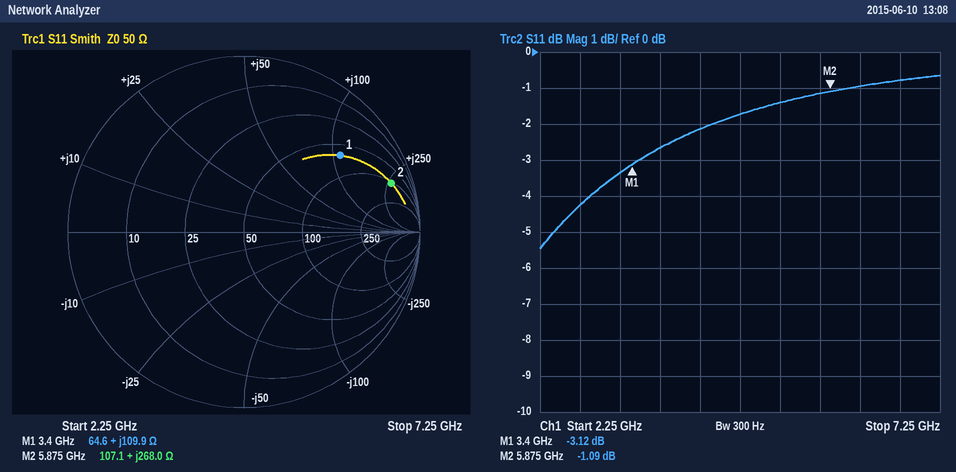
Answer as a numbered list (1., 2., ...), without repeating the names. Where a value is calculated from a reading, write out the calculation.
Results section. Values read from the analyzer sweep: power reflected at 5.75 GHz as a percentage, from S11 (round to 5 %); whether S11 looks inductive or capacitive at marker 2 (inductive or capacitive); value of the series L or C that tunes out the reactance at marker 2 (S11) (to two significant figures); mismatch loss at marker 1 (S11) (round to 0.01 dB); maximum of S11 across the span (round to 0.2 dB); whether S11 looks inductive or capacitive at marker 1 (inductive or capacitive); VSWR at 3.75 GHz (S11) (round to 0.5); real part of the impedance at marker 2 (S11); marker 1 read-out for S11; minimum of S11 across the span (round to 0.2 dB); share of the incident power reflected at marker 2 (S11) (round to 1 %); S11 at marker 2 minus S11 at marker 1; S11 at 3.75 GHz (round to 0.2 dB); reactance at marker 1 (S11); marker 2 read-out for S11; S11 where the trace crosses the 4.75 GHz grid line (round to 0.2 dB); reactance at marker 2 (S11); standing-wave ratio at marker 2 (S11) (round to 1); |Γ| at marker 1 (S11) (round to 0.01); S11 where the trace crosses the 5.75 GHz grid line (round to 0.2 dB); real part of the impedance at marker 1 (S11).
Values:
1. 10^(-1.2/10) ≈ 75.9 %, so 75 % to the nearest 5 %
2. inductive
3. C = 1/(2π × 5.875 GHz × 268 Ω) ≈ 101 fF, so 100 fF to two significant figures
4. −10 log10(1 − 10^(-3.12/10)) ≈ 2.90 dB
5. -0.6 dB
6. inductive
7. |Γ| = 10^(-2.6/20) = 0.7413; VSWR = (1 + 0.7413)/(1 − 0.7413) ≈ 6.73, so 6.5 to the nearest 0.5
8. 107.1 Ω
9. -3.12 dB
10. -5.4 dB
11. 10^(-1.09/10) ≈ 78 %
12. -1.09 − (-3.12) = 2.03 dB
13. -2.6 dB
14. +109.9 Ω
15. -1.09 dB
16. -1.8 dB
17. +268.0 Ω
18. 16
19. 0.70
20. -1.2 dB
21. 64.6 Ω
